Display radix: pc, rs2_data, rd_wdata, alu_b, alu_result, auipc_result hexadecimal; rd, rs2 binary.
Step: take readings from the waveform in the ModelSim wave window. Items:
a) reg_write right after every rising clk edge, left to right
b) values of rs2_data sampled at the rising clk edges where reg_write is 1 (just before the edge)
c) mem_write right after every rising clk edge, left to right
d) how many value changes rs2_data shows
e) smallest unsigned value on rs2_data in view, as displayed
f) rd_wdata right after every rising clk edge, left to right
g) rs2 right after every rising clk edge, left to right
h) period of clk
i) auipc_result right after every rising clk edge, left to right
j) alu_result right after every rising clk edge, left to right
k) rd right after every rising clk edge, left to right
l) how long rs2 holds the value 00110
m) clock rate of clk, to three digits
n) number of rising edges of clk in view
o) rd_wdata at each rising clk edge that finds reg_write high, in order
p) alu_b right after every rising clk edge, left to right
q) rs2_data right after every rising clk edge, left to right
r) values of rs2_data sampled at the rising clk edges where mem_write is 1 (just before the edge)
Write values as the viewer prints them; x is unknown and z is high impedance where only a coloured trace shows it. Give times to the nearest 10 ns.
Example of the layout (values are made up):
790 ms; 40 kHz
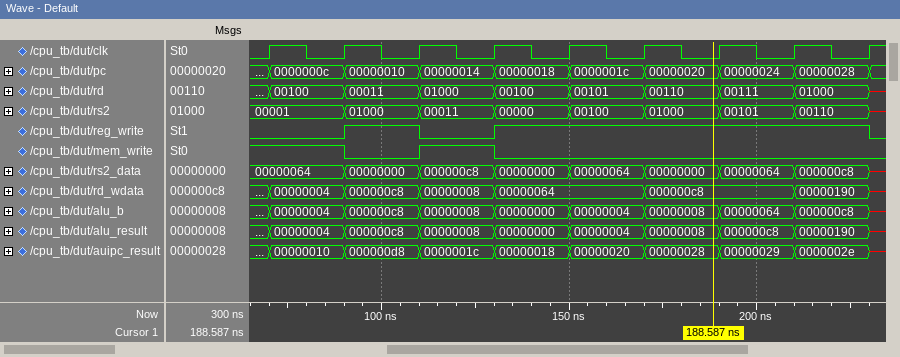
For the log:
0 1 0 1 1 1 1 1 0; 00000000, 00000000, 00000064, 00000000, 00000064, 000000c8; 1 0 1 0 0 0 0 0 0; 8; 00000000; 00000004, 000000c8, 00000008, 00000064, 00000064, 000000c8, 000000c8, 00000190, x; 00001, 01000, 00011, 00000, 00100, 01000, 00101, 00110, x; 20 ns; 00000010, 000000d8, 0000001c, 00000018, 00000020, 00000028, 00000029, 0000002e, x; 00000004, 000000c8, 00000008, 00000000, 00000004, 00000008, 000000c8, 00000190, x; 00100, 00011, 01000, 00100, 00101, 00110, 00111, 01000, x; 20 ns; 50.0 MHz; 9; 000000c8, 00000064, 00000064, 000000c8, 000000c8, 00000190; 00000004, 000000c8, 00000008, 00000000, 00000004, 00000008, 00000064, 000000c8, x; 00000064, 00000000, 000000c8, 00000000, 00000064, 00000000, 00000064, 000000c8, x; 00000064, 00000064, 000000c8
